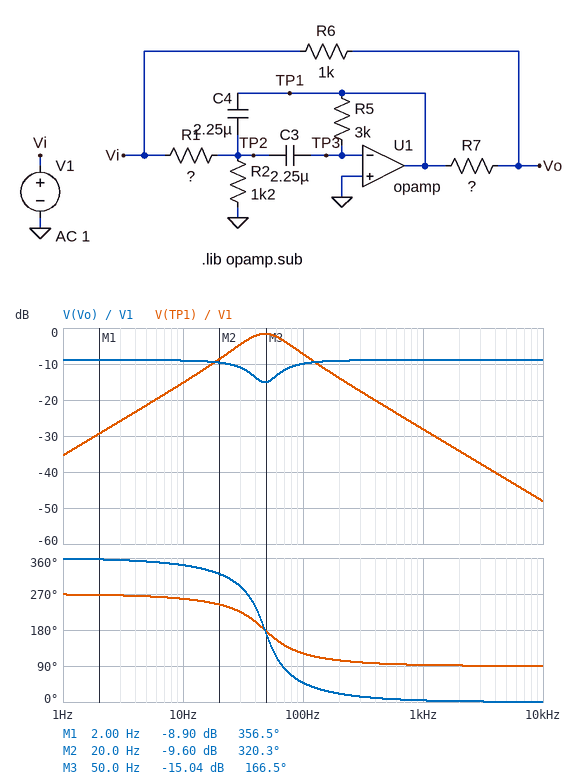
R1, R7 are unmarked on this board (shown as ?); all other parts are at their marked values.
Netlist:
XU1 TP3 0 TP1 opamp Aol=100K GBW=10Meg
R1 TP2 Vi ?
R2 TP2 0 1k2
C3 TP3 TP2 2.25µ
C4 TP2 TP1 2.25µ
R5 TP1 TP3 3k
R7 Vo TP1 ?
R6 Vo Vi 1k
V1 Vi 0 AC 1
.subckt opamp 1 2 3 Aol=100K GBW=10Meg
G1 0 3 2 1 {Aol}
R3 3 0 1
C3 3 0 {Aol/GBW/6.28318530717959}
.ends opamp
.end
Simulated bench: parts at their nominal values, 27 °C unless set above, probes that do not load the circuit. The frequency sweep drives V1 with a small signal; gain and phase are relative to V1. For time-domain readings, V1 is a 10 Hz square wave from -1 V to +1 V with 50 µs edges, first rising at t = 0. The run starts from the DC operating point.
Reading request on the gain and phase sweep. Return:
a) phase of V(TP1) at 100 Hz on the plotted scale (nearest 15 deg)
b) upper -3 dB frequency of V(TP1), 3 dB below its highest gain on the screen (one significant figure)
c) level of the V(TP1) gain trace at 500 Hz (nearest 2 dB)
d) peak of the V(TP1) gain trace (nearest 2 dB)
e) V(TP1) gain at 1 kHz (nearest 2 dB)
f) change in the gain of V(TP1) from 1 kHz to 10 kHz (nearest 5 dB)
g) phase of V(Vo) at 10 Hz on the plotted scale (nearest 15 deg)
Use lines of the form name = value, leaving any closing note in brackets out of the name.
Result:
phase of V(TP1) at 100 Hz on the plotted scale = 120 deg
upper -3 dB frequency of V(TP1), 3 dB below its highest gain on the screen = 80 Hz
level of the V(TP1) gain trace at 500 Hz = -22 dB
peak of the V(TP1) gain trace = -2 dB
V(TP1) gain at 1 kHz = -28 dB
change in the gain of V(TP1) from 1 kHz to 10 kHz = -20 dB
phase of V(Vo) at 10 Hz on the plotted scale = 345 deg
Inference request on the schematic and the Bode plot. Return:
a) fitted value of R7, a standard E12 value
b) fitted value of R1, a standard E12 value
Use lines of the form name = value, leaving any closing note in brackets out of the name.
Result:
fitted value of R7, a standard E12 value = 560 Ω
fitted value of R1, a standard E12 value = 1.8 kΩ
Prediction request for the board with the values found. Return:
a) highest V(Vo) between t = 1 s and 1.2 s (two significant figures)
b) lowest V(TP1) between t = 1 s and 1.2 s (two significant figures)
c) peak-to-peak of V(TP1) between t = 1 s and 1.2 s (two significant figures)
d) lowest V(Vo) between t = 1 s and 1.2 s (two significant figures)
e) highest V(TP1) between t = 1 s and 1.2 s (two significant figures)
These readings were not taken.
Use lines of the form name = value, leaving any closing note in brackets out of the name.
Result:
highest V(Vo) between t = 1 s and 1.2 s = 460 mV
lowest V(TP1) between t = 1 s and 1.2 s = -900 mV
peak-to-peak of V(TP1) between t = 1 s and 1.2 s = 1.8 V
lowest V(Vo) between t = 1 s and 1.2 s = -460 mV
highest V(TP1) between t = 1 s and 1.2 s = 900 mV
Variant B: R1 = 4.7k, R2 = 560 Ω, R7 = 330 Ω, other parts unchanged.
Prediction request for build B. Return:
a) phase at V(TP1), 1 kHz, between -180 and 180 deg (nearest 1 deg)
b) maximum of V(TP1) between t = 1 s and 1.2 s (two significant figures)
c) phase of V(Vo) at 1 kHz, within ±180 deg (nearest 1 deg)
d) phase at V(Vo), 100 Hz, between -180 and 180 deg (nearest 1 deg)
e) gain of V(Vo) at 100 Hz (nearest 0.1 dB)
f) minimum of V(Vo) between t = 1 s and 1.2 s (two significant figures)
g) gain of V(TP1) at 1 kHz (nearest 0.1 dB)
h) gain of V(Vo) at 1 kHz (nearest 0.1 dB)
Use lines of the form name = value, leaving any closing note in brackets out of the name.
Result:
phase at V(TP1), 1 kHz, between -180 and 180 deg = 93 deg
maximum of V(TP1) between t = 1 s and 1.2 s = 310 mV
phase of V(Vo) at 1 kHz, within ±180 deg = 3 deg
phase at V(Vo), 100 Hz, between -180 and 180 deg = 34 deg
gain of V(Vo) at 100 Hz = -13.9 dB
minimum of V(Vo) between t = 1 s and 1.2 s = -310 mV
gain of V(TP1) at 1 kHz = -36.4 dB
gain of V(Vo) at 1 kHz = -12.1 dB
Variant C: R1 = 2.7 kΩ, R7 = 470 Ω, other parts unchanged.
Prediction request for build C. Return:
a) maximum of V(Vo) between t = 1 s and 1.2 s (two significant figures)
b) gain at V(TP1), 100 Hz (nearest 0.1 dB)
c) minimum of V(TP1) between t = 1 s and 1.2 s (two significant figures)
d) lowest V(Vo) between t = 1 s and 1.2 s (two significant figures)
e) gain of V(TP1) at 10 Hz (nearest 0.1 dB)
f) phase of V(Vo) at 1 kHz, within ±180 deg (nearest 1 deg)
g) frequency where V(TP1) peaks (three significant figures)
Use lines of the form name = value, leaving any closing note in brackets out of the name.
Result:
maximum of V(Vo) between t = 1 s and 1.2 s = 380 mV
gain at V(TP1), 100 Hz = -11.0 dB
minimum of V(TP1) between t = 1 s and 1.2 s = -620 mV
lowest V(Vo) between t = 1 s and 1.2 s = -380 mV
gain of V(TP1) at 10 Hz = -17.5 dB
phase of V(Vo) at 1 kHz, within ±180 deg = 3 deg
frequency where V(TP1) peaks = 44.8 Hz
